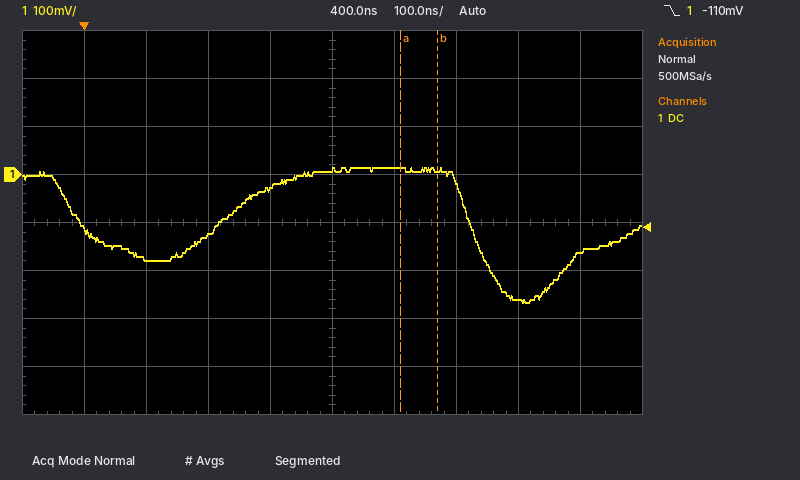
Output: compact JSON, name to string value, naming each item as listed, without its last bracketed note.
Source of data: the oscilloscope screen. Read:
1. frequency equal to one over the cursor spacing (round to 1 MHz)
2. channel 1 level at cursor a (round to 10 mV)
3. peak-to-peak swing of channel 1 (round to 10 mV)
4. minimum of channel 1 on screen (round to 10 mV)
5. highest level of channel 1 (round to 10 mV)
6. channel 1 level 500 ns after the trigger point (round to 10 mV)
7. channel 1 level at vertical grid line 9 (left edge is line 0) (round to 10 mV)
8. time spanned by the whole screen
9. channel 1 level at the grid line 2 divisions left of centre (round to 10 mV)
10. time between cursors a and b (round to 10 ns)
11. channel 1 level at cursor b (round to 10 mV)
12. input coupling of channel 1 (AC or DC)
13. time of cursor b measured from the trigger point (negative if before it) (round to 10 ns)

{"frequency equal to one over the cursor spacing": "17 MHz", "channel 1 level at cursor a": "10 mV", "peak-to-peak swing of channel 1": "280 mV", "minimum of channel 1 on screen": "-270 mV", "highest level of channel 1": "10 mV", "channel 1 level 500 ns after the trigger point": "10 mV", "channel 1 level at vertical grid line 9 (left edge is line 0)": "-160 mV", "time spanned by the whole screen": "1 µs", "channel 1 level at the grid line 2 divisions left of centre": "-130 mV", "time between cursors a and b": "60 ns", "channel 1 level at cursor b": "10 mV", "input coupling of channel 1": "DC", "time of cursor b measured from the trigger point (negative if before it)": "+570 ns"}
